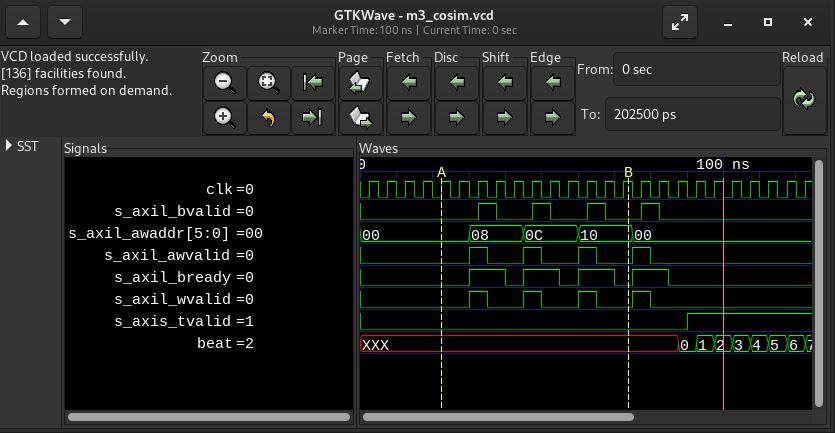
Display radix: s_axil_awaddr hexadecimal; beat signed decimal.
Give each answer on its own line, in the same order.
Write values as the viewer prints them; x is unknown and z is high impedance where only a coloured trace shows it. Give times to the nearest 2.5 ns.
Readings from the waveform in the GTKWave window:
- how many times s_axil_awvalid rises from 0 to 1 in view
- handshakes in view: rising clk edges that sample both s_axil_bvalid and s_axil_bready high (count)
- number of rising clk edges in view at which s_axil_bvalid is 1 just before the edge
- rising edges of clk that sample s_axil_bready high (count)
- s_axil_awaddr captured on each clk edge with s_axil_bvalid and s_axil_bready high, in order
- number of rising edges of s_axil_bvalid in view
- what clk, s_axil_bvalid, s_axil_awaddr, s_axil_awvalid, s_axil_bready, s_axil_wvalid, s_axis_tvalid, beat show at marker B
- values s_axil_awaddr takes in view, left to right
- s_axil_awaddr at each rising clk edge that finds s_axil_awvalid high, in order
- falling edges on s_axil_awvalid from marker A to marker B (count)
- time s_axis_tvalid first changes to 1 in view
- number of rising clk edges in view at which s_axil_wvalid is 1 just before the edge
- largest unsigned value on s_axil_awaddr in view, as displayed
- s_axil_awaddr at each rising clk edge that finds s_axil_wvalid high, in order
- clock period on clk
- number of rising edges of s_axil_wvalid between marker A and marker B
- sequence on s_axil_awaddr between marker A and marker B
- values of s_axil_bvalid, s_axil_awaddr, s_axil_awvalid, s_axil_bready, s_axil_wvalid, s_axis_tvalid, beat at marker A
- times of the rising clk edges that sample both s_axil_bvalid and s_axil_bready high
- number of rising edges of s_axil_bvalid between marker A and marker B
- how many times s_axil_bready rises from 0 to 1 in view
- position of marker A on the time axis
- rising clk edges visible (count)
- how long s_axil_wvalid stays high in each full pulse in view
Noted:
4
4
4
8
08, 0C, 10, 00
4
clk=1, s_axil_bvalid=0, s_axil_awaddr=10, s_axil_awvalid=0, s_axil_bready=0, s_axil_wvalid=0, s_axis_tvalid=0, beat=XXX
00, 08, 0C, 10, 00
08, 0C, 10, 00
3
90 ns
4
10
08, 0C, 10, 00
5 ns
3
00, 08, 0C, 10
s_axil_bvalid=0, s_axil_awaddr=00, s_axil_awvalid=0, s_axil_bready=0, s_axil_wvalid=0, s_axis_tvalid=0, beat=XXX
37.5 ns, 52.5 ns, 67.5 ns, 82.5 ns
3
4
22.5 ns
25
5 ns, 5 ns, 5 ns, 5 ns
